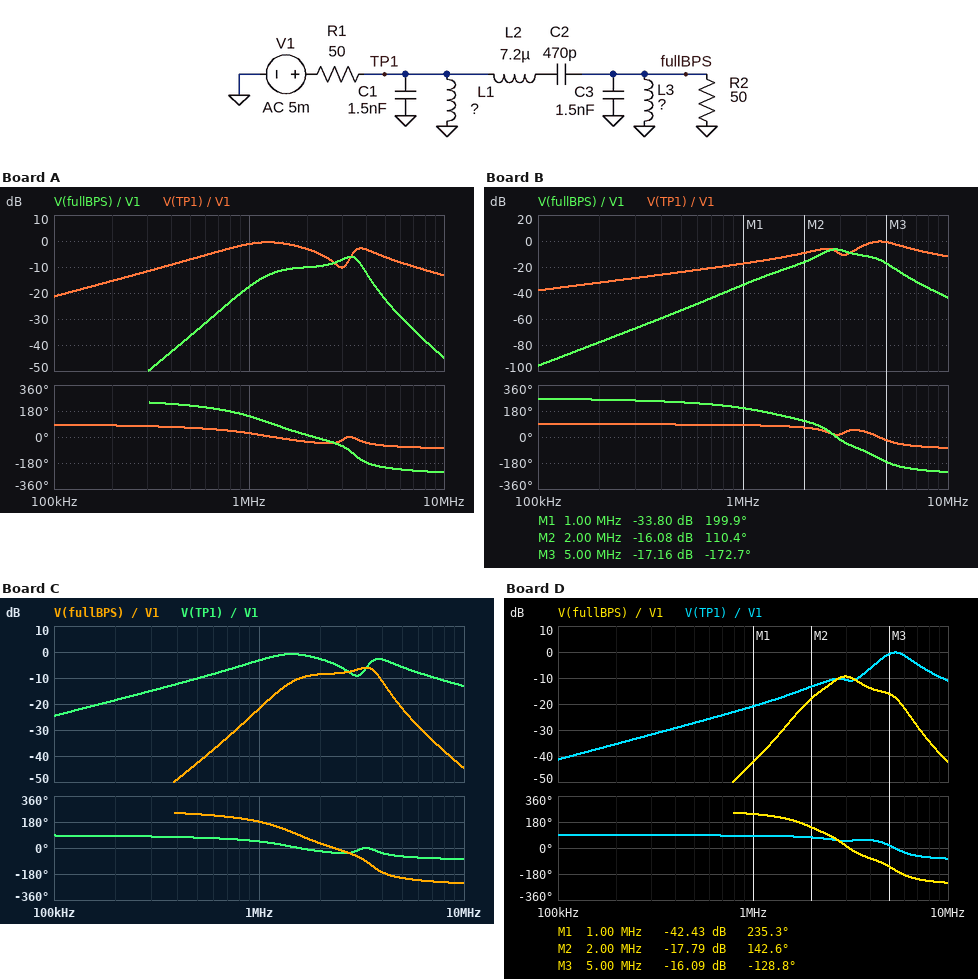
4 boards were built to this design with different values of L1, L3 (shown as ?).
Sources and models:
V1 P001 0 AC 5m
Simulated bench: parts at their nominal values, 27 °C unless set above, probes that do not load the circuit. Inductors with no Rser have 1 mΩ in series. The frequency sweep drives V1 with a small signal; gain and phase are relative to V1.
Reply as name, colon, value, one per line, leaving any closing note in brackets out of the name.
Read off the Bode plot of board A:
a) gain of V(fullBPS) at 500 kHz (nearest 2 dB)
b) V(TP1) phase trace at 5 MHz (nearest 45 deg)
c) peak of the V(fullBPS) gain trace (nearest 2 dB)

gain of V(fullBPS) at 500 kHz: -36 dB
V(TP1) phase trace at 5 MHz: -45 deg
peak of the V(fullBPS) gain trace: -6 dB
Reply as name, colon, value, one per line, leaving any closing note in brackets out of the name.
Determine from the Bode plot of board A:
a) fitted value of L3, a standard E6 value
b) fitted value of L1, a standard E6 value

fitted value of L3, a standard E6 value: 6.8 µH
fitted value of L1, a standard E6 value: 6.8 µH
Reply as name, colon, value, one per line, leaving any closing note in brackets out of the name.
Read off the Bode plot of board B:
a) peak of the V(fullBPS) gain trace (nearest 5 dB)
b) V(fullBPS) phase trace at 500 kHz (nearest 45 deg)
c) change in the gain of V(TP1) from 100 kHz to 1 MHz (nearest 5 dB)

peak of the V(fullBPS) gain trace: -5 dB
V(fullBPS) phase trace at 500 kHz: 225 deg
change in the gain of V(TP1) from 100 kHz to 1 MHz: 20 dB
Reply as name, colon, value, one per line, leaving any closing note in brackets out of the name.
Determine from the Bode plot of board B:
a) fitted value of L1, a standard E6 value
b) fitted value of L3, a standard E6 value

fitted value of L1, a standard E6 value: 1 µH
fitted value of L3, a standard E6 value: 6.8 µH
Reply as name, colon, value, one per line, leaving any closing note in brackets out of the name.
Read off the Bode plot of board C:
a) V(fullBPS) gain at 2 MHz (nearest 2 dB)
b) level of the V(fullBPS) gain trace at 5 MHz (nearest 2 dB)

V(fullBPS) gain at 2 MHz: -8 dB
level of the V(fullBPS) gain trace at 5 MHz: -22 dB
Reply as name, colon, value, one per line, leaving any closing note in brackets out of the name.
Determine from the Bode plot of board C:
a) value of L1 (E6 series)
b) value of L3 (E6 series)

value of L1: 4.7 µH
value of L3: 4.7 µH
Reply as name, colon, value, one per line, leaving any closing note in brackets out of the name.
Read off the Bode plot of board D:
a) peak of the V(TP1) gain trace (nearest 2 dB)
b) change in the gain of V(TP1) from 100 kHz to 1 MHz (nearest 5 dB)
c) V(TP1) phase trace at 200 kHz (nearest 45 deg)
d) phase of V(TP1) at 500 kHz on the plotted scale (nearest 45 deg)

peak of the V(TP1) gain trace: 0 dB
change in the gain of V(TP1) from 100 kHz to 1 MHz: 20 dB
V(TP1) phase trace at 200 kHz: 90 deg
phase of V(TP1) at 500 kHz on the plotted scale: 90 deg
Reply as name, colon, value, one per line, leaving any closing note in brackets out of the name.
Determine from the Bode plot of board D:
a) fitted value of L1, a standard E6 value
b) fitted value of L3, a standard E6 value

fitted value of L1, a standard E6 value: 680 nH
fitted value of L3, a standard E6 value: 3.3 µH
